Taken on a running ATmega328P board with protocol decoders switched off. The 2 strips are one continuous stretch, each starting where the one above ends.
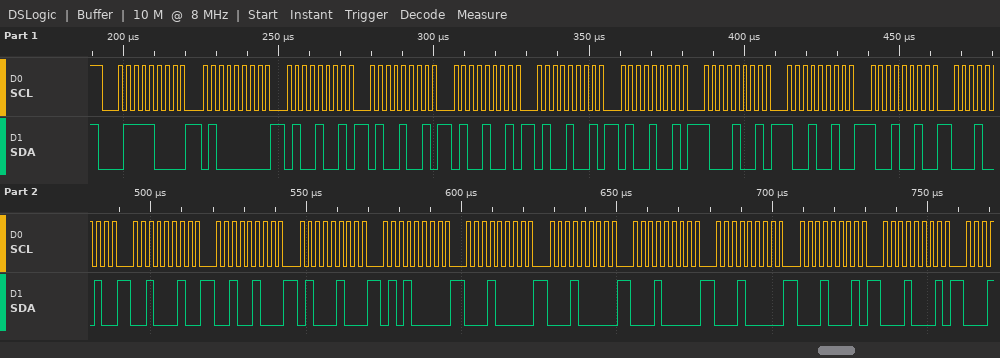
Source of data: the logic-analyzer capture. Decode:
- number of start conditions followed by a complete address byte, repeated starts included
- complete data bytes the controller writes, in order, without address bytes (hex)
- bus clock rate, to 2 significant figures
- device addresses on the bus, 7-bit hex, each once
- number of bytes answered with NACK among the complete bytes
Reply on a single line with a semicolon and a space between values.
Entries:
1; 40 49 49 49 49 49 89 92 92 12 22 24 44 50 10 10 10 10 11 11; 400 kHz; 0x3C; 0
